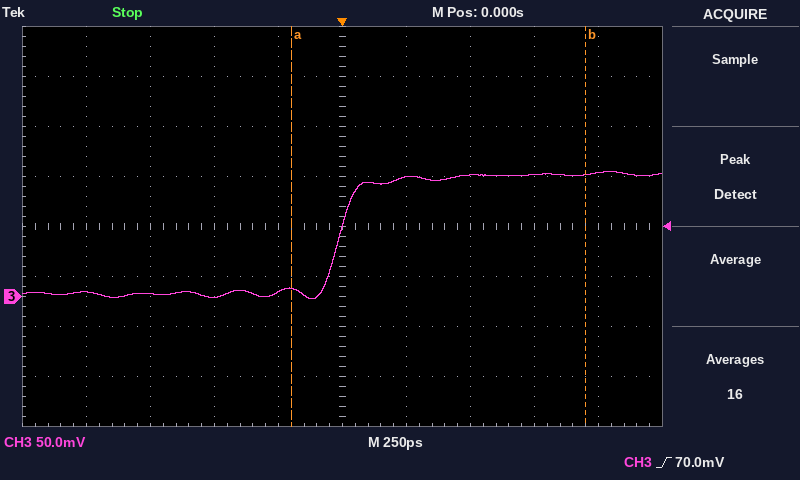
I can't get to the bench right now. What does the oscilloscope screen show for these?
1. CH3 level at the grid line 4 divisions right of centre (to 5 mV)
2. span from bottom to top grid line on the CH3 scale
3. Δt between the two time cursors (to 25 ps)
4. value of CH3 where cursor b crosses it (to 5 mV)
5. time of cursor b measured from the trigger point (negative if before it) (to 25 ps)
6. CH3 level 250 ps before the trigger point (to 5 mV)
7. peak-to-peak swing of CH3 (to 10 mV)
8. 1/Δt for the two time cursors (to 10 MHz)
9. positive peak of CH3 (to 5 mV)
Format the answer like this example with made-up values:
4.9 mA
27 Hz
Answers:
125 mV
400 mV
1.150 ns
120 mV
+950 ps
5 mV
130 mV
870 MHz
125 mV
